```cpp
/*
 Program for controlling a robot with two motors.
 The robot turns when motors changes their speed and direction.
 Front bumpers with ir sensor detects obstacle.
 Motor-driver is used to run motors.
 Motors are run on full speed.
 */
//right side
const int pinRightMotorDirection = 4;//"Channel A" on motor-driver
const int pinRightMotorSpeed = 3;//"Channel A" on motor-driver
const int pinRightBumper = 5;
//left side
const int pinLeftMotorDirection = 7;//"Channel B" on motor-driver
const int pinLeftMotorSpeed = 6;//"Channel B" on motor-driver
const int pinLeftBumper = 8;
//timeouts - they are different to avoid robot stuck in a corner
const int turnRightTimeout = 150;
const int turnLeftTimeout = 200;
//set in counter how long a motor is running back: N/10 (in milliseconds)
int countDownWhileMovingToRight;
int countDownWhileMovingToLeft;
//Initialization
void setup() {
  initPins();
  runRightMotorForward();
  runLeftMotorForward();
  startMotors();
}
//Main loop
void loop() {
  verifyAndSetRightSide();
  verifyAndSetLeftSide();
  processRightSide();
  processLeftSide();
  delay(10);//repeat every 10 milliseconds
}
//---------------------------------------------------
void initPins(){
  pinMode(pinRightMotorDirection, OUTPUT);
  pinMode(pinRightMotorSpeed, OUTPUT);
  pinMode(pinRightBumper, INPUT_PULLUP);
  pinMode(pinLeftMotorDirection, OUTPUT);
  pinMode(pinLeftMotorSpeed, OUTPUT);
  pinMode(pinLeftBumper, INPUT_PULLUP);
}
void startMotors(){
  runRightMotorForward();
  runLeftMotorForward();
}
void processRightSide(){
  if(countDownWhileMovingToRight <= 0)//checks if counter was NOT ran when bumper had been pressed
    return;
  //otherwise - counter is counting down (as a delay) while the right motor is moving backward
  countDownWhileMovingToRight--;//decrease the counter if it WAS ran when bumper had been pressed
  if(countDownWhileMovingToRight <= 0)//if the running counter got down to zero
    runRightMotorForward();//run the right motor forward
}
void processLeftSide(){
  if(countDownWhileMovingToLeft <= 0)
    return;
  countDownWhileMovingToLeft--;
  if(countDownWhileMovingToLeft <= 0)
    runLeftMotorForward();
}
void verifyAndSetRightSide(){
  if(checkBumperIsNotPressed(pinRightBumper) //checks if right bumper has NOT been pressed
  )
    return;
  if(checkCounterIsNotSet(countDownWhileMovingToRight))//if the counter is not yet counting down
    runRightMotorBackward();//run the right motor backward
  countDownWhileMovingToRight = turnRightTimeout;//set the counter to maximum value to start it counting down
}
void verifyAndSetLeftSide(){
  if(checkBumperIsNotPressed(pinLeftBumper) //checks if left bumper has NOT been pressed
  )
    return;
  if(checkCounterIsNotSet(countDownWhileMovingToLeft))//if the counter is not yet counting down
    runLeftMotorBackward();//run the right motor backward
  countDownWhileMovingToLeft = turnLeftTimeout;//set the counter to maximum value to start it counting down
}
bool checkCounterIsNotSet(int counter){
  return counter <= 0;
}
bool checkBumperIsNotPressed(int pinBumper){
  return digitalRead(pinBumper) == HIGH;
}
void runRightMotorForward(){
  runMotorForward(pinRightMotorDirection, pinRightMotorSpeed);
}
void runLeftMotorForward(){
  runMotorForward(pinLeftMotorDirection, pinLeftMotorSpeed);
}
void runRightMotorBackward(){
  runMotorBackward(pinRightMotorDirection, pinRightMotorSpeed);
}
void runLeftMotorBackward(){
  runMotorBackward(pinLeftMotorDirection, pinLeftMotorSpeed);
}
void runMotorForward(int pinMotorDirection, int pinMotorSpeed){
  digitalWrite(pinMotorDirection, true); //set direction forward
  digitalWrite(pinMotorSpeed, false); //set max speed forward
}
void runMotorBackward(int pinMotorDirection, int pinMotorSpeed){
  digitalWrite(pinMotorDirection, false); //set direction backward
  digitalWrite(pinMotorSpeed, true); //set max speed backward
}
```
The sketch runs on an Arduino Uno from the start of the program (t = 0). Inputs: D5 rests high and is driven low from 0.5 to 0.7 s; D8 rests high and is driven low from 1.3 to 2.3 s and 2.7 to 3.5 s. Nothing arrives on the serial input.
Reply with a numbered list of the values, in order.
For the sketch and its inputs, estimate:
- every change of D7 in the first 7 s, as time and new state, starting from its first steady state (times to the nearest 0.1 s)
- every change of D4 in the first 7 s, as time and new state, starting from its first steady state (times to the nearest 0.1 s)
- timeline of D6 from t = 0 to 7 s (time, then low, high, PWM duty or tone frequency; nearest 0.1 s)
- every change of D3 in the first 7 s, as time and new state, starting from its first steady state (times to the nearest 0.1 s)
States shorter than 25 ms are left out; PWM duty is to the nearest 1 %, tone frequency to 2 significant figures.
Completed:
1. 0 s high; 1.3 s low; 5.5 s high
2. 0 s high; 0.5 s low; 2.2 s high
3. 0 s low; 1.3 s high; 5.5 s low
4. 0 s low; 0.5 s high; 2.2 s low
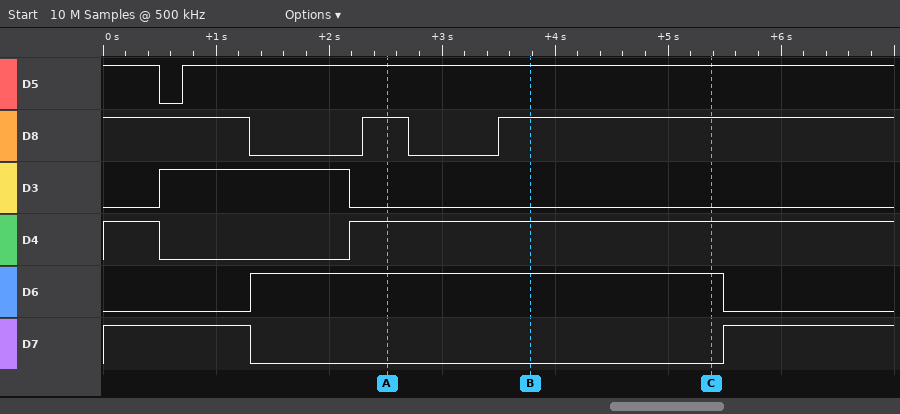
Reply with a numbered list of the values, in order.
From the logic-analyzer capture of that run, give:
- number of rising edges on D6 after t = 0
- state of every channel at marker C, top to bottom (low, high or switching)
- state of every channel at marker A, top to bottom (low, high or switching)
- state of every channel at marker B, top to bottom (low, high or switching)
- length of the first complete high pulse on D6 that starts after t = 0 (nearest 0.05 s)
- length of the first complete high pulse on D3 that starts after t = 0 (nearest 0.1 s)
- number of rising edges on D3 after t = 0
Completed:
1. 1
2. D5 high, D8 high, D3 low, D4 high, D6 high, D7 low
3. D5 high, D8 high, D3 low, D4 high, D6 high, D7 low
4. D5 high, D8 high, D3 low, D4 high, D6 high, D7 low
5. 4.20 s
6. 1.7 s
7. 1
